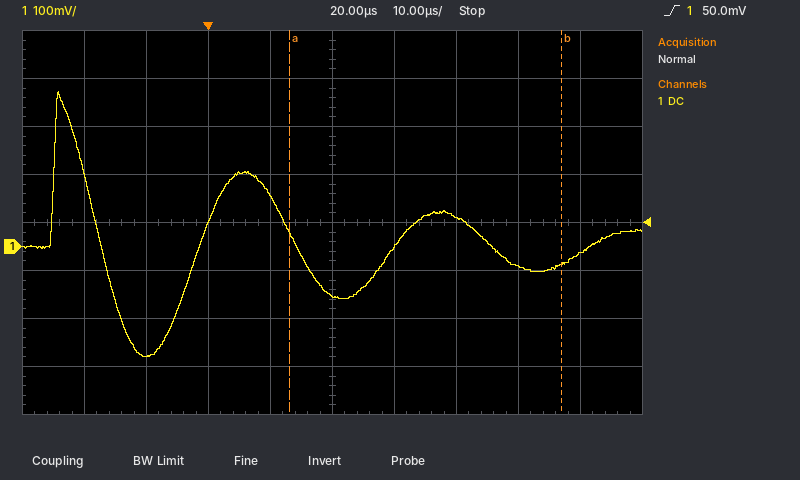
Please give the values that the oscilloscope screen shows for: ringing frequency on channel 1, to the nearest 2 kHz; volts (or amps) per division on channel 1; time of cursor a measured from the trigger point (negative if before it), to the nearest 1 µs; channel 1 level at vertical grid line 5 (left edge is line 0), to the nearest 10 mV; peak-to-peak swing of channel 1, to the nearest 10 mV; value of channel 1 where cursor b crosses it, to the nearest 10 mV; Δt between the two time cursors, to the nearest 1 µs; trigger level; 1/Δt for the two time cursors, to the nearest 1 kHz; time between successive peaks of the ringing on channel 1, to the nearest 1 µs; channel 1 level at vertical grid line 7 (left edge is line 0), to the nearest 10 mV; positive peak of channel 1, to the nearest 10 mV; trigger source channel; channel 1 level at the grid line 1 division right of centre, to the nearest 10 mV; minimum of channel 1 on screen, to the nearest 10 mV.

32 kHz
100 mV
+13 µs
-100 mV
550 mV
-40 mV
44 µs
50.0 mV
23 kHz
31 µs
60 mV
320 mV
channel 1
0 mV
-230 mV
